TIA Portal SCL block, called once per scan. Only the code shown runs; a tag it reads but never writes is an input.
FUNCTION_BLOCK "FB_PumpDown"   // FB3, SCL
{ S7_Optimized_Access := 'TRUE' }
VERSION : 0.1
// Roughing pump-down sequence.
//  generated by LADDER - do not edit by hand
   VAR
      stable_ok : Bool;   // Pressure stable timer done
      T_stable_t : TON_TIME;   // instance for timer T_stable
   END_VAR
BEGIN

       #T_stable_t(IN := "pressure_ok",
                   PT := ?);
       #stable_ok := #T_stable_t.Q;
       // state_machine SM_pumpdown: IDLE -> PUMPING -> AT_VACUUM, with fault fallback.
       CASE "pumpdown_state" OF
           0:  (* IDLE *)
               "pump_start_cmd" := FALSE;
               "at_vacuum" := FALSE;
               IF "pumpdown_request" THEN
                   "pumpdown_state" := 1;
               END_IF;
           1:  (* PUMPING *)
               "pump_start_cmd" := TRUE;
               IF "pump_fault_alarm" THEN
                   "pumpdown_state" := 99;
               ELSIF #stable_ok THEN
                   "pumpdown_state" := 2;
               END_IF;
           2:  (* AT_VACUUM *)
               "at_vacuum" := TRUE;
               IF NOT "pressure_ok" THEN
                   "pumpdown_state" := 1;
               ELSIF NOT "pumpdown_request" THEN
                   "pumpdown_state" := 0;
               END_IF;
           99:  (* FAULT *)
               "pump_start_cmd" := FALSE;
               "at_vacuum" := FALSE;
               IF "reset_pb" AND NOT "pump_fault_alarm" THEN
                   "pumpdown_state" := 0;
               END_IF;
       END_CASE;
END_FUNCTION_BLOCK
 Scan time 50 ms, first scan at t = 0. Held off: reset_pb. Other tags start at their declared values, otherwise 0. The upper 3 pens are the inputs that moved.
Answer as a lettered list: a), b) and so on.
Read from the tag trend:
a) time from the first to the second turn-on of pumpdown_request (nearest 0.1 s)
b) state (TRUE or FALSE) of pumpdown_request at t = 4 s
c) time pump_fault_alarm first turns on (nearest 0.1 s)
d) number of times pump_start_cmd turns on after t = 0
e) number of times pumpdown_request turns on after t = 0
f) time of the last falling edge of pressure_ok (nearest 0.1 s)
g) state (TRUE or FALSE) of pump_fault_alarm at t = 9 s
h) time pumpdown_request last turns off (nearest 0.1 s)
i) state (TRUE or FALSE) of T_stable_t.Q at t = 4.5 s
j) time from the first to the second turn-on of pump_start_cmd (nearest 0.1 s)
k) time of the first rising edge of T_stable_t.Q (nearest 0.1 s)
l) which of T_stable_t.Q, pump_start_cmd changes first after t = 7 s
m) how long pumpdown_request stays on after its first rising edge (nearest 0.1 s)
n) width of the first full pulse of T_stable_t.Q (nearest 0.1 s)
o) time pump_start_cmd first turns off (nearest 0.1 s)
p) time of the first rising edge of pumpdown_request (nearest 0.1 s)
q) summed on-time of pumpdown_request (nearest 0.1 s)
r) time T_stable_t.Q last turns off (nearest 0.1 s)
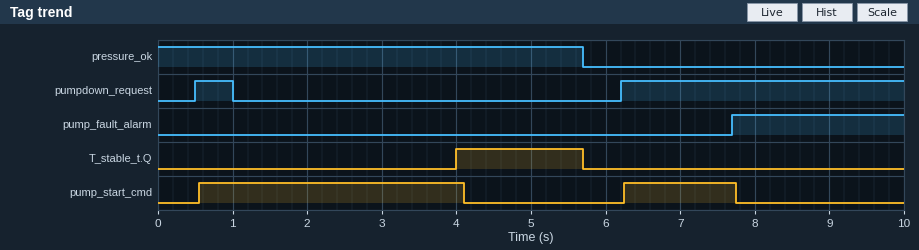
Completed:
a) 5.7 s
b) FALSE
c) 7.7 s
d) 2
e) 2
f) 5.7 s
g) TRUE
h) 1.0 s
i) TRUE
j) 5.7 s
k) 4.0 s
l) pump_start_cmd
m) 0.5 s
n) 1.7 s
o) 4.1 s
p) 0.5 s
q) 4.3 s
r) 5.7 s
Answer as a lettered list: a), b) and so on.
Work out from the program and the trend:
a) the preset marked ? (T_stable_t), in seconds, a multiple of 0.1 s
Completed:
a) 4.0 s
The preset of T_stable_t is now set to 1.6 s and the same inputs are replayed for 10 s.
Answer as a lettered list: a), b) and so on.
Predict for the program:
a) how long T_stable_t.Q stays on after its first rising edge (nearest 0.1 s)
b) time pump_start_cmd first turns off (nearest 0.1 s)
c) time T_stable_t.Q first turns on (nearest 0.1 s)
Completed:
a) 4.1 s
b) 1.7 s
c) 1.6 s
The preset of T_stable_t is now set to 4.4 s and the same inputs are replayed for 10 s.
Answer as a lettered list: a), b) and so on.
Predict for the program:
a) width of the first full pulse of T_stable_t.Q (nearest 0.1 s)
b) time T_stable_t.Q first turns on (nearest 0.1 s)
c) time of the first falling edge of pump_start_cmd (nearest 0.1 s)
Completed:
a) 1.3 s
b) 4.4 s
c) 4.5 s
